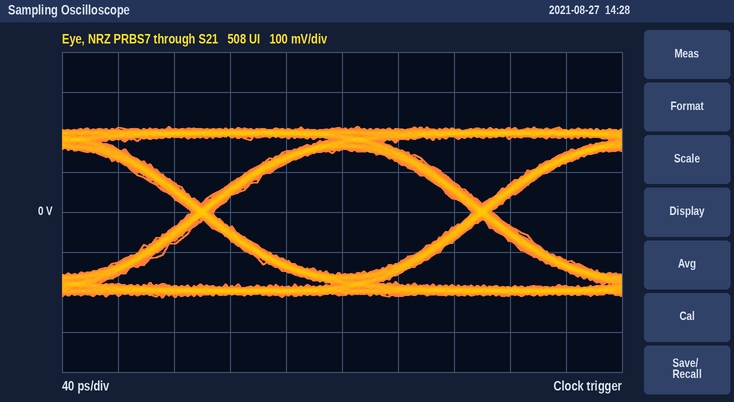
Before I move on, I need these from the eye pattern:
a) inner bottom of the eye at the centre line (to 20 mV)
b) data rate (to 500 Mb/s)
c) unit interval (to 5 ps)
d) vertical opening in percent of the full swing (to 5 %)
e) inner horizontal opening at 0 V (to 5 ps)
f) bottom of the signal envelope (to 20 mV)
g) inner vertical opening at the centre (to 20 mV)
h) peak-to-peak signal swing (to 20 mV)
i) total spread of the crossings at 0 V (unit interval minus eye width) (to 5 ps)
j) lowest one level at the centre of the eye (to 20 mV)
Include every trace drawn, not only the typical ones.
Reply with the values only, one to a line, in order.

-160 mV
5.0 Gb/s
200 ps
75 %
185 ps
-220 mV
320 mV
420 mV
15 ps
160 mV
